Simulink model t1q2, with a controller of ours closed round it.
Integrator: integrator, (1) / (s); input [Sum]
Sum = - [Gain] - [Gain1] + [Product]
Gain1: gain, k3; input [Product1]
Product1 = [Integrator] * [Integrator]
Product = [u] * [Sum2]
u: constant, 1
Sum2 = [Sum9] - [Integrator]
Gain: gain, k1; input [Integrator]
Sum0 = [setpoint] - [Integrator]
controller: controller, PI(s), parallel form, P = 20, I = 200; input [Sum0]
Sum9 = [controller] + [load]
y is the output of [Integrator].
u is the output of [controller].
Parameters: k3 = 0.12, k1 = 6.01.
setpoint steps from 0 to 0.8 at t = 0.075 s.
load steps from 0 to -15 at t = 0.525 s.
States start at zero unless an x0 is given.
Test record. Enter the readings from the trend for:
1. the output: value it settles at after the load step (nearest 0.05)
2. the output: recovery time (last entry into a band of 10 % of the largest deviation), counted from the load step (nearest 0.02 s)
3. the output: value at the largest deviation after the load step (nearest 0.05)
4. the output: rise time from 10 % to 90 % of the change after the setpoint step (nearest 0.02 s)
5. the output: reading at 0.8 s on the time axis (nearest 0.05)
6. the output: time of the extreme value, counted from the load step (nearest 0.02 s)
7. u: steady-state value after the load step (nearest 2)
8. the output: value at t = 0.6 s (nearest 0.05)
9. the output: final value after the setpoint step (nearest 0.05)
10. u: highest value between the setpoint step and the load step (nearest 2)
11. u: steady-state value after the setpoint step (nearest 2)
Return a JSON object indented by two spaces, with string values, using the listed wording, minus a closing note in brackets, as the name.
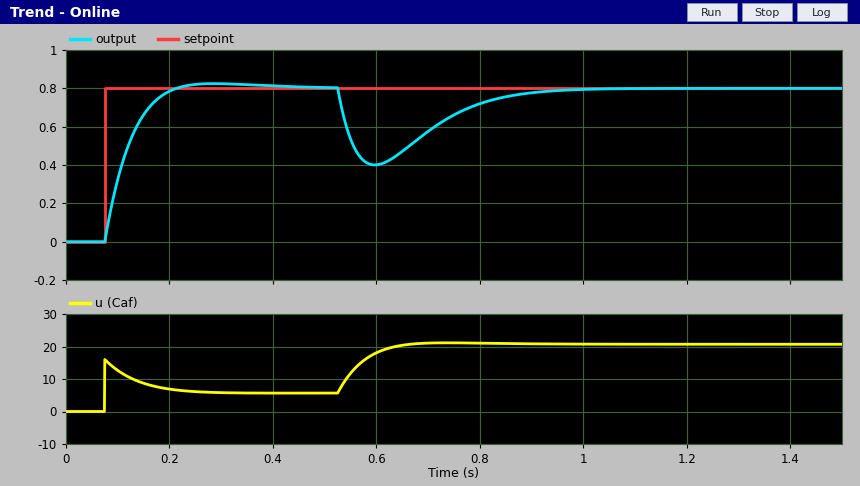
{
  "the output: value it settles at after the load step": "0.80",
  "the output: recovery time (last entry into a band of 10 % of the largest deviation), counted from the load step": "0.34 s",
  "the output: value at the largest deviation after the load step": "0.40",
  "the output: rise time from 10 % to 90 % of the change after the setpoint step": "0.08 s",
  "the output: reading at 0.8 s on the time axis": "0.70",
  "the output: time of the extreme value, counted from the load step": "0.08 s",
  "u: steady-state value after the load step": "20",
  "the output: value at t = 0.6 s": "0.40",
  "the output: final value after the setpoint step": "0.80",
  "u: highest value between the setpoint step and the load step": "16",
  "u: steady-state value after the setpoint step": "6"
}
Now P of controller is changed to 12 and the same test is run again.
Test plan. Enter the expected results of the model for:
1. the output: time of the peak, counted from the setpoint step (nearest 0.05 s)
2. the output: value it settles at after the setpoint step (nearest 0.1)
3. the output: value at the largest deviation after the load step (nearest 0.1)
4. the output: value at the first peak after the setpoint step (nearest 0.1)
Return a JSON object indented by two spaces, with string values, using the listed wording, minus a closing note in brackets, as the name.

{
  "the output: time of the peak, counted from the setpoint step": "0.20 s",
  "the output: value it settles at after the setpoint step": "0.8",
  "the output: value at the largest deviation after the load step": "0.3",
  "the output: value at the first peak after the setpoint step": "0.9"
}
